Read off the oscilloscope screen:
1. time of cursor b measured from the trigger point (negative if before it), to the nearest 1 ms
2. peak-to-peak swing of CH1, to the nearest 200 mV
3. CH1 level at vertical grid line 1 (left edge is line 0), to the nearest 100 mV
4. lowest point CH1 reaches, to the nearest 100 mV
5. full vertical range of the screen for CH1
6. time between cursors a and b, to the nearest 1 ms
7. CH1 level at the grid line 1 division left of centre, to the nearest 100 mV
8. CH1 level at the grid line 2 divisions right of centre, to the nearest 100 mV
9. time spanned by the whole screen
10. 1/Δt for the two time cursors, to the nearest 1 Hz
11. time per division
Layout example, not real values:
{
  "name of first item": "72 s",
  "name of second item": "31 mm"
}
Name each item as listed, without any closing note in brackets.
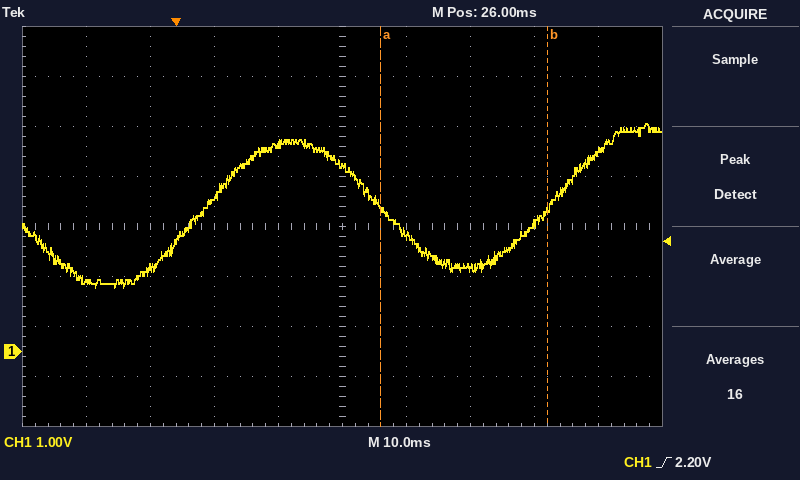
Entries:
{
  "time of cursor b measured from the trigger point (negative if before it), to the nearest 1 ms": "+58 ms",
  "peak-to-peak swing of CH1, to the nearest 200 mV": "3.2 V",
  "CH1 level at vertical grid line 1 (left edge is line 0), to the nearest 100 mV": "1.4 V",
  "lowest point CH1 reaches, to the nearest 100 mV": "1.3 V",
  "full vertical range of the screen for CH1": "8 V",
  "time between cursors a and b, to the nearest 1 ms": "26 ms",
  "CH1 level at the grid line 1 division left of centre, to the nearest 100 mV": "4.2 V",
  "CH1 level at the grid line 2 divisions right of centre, to the nearest 100 mV": "1.7 V",
  "time spanned by the whole screen": "100 ms",
  "1/Δt for the two time cursors, to the nearest 1 Hz": "38 Hz",
  "time per division": "10 ms"
}
